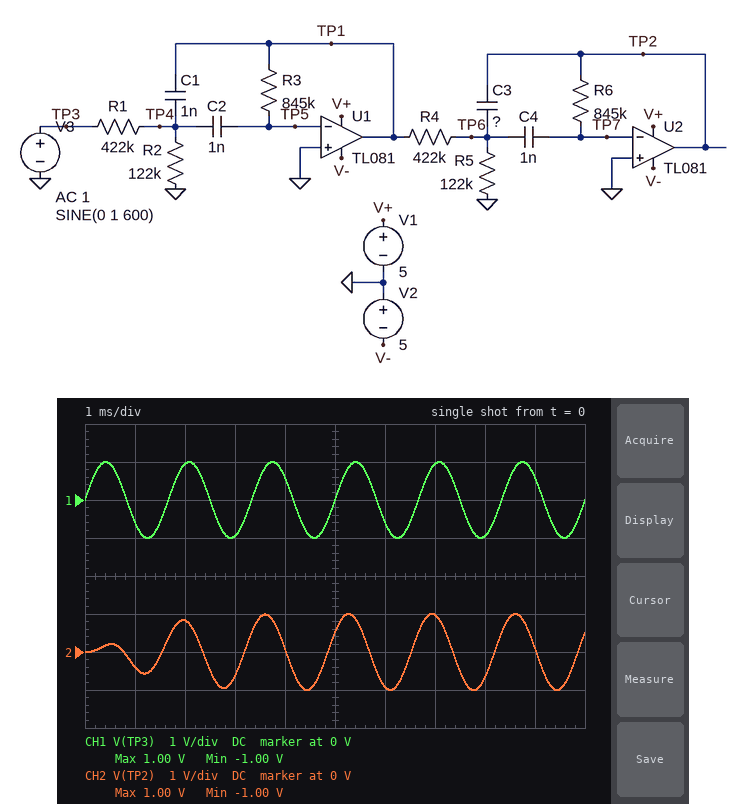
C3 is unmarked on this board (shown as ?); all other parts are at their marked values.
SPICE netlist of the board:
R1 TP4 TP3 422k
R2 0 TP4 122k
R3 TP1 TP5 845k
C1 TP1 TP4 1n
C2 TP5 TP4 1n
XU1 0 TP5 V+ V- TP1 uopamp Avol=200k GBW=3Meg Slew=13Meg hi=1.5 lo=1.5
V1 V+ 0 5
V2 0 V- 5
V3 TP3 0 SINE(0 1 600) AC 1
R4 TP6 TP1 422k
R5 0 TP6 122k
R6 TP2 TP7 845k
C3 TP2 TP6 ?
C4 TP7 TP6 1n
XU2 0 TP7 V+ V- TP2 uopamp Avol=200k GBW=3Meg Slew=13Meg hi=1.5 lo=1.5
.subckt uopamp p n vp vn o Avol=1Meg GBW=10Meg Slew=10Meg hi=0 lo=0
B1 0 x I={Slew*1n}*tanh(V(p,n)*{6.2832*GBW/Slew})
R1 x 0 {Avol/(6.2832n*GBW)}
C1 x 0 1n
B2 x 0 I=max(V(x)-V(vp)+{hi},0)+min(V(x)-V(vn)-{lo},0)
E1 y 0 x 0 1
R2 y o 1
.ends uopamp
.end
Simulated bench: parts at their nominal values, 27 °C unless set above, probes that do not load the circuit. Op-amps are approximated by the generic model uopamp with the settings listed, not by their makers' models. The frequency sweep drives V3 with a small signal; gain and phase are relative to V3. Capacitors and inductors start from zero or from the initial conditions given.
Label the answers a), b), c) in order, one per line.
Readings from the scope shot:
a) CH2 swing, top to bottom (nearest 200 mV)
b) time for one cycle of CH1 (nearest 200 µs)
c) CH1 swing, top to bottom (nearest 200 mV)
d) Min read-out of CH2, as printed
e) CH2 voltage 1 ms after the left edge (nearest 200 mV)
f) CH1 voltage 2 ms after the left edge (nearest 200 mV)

a) 2.0 V
b) 1.6 ms
c) 2.0 V
d) -1.00 V
e) -400 mV
f) 1.0 V
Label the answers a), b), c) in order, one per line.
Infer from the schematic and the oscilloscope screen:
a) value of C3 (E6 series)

a) 470 pF
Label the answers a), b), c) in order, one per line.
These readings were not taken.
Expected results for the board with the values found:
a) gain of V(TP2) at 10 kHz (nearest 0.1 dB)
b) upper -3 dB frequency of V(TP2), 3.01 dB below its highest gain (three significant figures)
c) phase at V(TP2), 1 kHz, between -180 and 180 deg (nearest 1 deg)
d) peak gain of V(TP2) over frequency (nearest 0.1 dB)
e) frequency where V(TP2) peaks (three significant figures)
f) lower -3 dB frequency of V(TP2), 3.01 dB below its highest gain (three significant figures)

a) -50.3 dB
b) 903 Hz
c) -90 deg
d) 0.4 dB
e) 668 Hz
f) 502 Hz
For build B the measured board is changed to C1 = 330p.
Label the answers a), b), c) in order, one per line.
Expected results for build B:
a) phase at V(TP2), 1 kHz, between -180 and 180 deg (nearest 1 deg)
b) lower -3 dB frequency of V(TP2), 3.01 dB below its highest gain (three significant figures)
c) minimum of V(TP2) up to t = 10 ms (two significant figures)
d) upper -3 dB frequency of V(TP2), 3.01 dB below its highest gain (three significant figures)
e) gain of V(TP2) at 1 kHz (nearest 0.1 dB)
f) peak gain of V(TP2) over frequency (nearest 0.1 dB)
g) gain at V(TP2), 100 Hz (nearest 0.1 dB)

a) -32 deg
b) 693 Hz
c) -970 mV
d) 1.15 kHz
e) 5.1 dB
f) 5.8 dB
g) -36.8 dB
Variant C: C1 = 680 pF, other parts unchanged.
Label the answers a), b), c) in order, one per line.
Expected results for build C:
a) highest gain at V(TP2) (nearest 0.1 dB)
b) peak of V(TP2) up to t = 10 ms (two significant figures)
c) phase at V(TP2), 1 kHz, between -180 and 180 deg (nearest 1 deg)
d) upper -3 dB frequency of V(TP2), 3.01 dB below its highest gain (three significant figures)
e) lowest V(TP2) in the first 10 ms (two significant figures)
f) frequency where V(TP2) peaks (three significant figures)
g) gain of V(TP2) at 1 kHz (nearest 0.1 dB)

a) 3.6 dB
b) 1.1 V
c) -78 deg
d) 948 Hz
e) -1.1 V
f) 744 Hz
g) -0.6 dB
